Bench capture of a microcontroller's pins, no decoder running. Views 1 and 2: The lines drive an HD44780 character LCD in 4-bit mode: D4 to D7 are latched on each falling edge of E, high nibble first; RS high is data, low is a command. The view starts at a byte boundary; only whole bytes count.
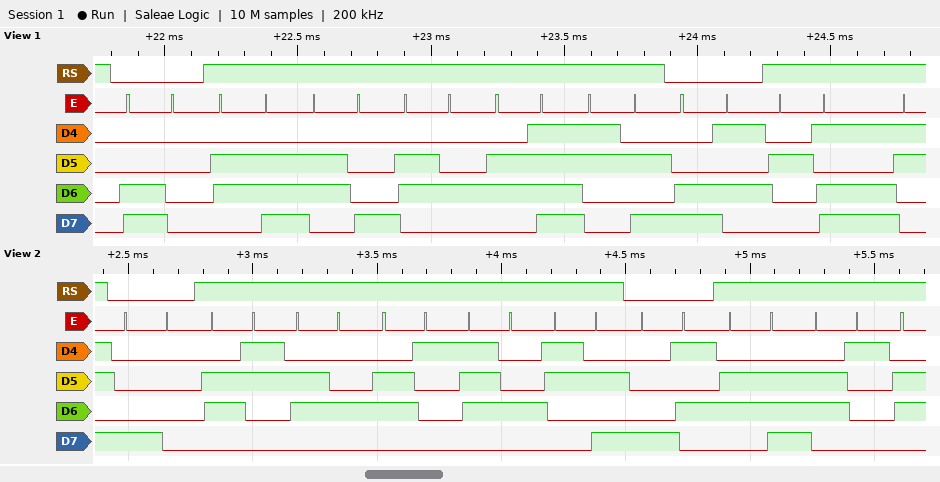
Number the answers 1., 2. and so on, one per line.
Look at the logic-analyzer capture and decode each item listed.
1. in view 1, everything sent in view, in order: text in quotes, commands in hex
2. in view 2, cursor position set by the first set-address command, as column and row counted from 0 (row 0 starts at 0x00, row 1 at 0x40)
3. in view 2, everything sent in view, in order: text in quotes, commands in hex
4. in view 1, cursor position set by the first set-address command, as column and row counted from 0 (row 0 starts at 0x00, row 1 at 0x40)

1. 0xC0 "nhdo:" 0xC5 "-"
2. column 0, row 0
3. 0x80 "cdat:" 0x85 "na"
4. column 0, row 1
